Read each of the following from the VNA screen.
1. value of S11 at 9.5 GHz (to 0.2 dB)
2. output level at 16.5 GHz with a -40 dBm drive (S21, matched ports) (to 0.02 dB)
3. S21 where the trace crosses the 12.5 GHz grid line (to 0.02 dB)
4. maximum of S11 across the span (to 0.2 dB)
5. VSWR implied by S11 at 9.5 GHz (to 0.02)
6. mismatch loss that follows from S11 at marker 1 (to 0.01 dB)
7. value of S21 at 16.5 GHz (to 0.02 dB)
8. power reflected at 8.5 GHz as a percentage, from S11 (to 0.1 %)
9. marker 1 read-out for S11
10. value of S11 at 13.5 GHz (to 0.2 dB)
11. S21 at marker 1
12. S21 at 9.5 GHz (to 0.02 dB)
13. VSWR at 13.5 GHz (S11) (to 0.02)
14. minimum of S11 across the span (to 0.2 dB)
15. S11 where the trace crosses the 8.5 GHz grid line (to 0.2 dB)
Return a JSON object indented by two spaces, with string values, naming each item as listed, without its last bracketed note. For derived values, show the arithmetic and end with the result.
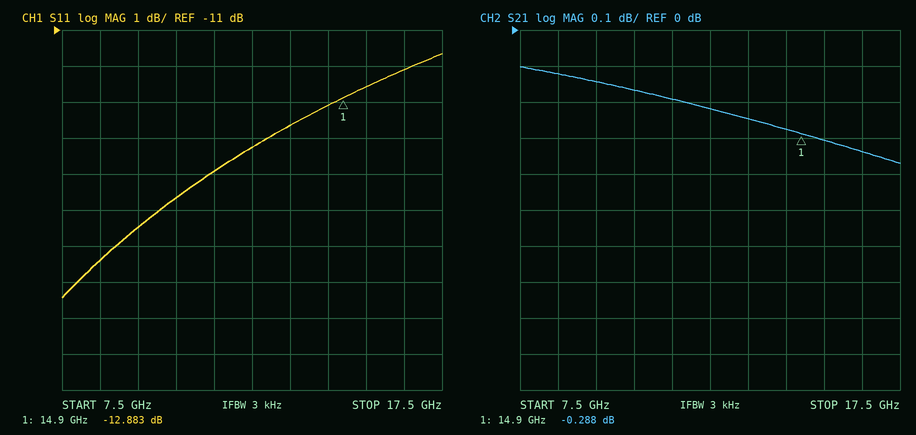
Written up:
{
  "value of S11 at 9.5 GHz": "-16.4 dB",
  "output level at 16.5 GHz with a -40 dBm drive (S21, matched ports)": "-40 dBm + (-0.34 dB) = -40.34 dBm",
  "S21 where the trace crosses the 12.5 GHz grid line": "-0.22 dB",
  "maximum of S11 across the span": "-11.6 dB",
  "VSWR implied by S11 at 9.5 GHz": "|Γ| = 10^(-16.4/20) = 0.1514; VSWR = (1 + 0.1514)/(1 − 0.1514) ≈ 1.36",
  "mismatch loss that follows from S11 at marker 1": "−10 log10(1 − 10^(-12.883/10)) ≈ 0.23 dB",
  "value of S21 at 16.5 GHz": "-0.34 dB",
  "power reflected at 8.5 GHz as a percentage, from S11": "10^(-17.4/10) ≈ 1.8 %",
  "marker 1 read-out for S11": "-12.883 dB",
  "value of S11 at 13.5 GHz": "-13.6 dB",
  "S21 at marker 1": "-0.288 dB",
  "S21 at 9.5 GHz": "-0.14 dB",
  "VSWR at 13.5 GHz (S11)": "|Γ| = 10^(-13.6/20) = 0.2089; VSWR = (1 + 0.2089)/(1 − 0.2089) ≈ 1.53, so 1.52 to the nearest 0.02",
  "minimum of S11 across the span": "-18.4 dB",
  "S11 where the trace crosses the 8.5 GHz grid line": "-17.4 dB"
}
